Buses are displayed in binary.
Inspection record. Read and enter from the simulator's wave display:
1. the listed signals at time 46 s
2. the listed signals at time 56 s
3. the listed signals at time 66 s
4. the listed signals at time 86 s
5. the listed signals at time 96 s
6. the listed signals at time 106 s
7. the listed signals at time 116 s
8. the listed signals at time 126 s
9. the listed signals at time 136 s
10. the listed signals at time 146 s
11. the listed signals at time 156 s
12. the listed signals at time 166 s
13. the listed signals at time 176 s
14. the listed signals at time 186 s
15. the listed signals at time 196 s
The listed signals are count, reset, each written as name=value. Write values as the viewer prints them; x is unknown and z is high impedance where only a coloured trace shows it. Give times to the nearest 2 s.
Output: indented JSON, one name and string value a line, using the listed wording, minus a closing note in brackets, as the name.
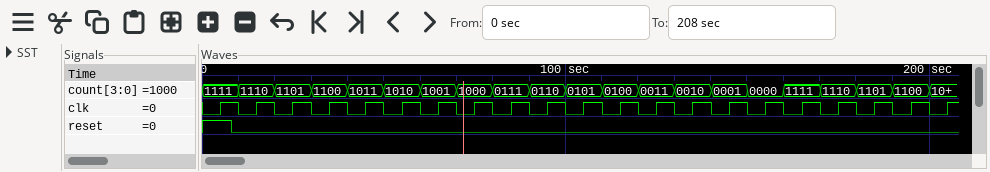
{
  "the listed signals at time 46 s": "count=1011, reset=0",
  "the listed signals at time 56 s": "count=1010, reset=0",
  "the listed signals at time 66 s": "count=1001, reset=0",
  "the listed signals at time 86 s": "count=0111, reset=0",
  "the listed signals at time 96 s": "count=0110, reset=0",
  "the listed signals at time 106 s": "count=0101, reset=0",
  "the listed signals at time 116 s": "count=0100, reset=0",
  "the listed signals at time 126 s": "count=0011, reset=0",
  "the listed signals at time 136 s": "count=0010, reset=0",
  "the listed signals at time 146 s": "count=0001, reset=0",
  "the listed signals at time 156 s": "count=0000, reset=0",
  "the listed signals at time 166 s": "count=1111, reset=0",
  "the listed signals at time 176 s": "count=1110, reset=0",
  "the listed signals at time 186 s": "count=1101, reset=0",
  "the listed signals at time 196 s": "count=1100, reset=0"
}
